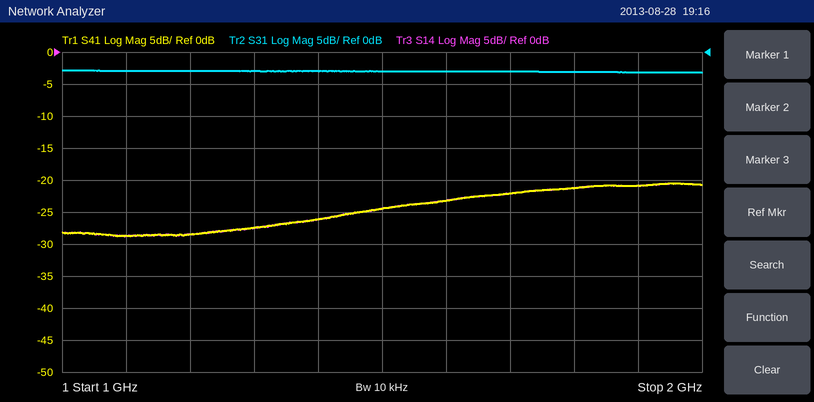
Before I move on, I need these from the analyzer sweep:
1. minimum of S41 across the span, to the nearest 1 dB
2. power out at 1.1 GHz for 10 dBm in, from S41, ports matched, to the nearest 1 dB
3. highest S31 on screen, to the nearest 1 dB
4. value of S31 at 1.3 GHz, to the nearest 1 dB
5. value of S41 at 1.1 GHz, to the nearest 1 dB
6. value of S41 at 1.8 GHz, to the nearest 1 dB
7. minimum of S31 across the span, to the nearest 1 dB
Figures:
-29 dB
-19 dBm
-3 dB
-3 dB
-29 dB
-21 dB
-3 dB
